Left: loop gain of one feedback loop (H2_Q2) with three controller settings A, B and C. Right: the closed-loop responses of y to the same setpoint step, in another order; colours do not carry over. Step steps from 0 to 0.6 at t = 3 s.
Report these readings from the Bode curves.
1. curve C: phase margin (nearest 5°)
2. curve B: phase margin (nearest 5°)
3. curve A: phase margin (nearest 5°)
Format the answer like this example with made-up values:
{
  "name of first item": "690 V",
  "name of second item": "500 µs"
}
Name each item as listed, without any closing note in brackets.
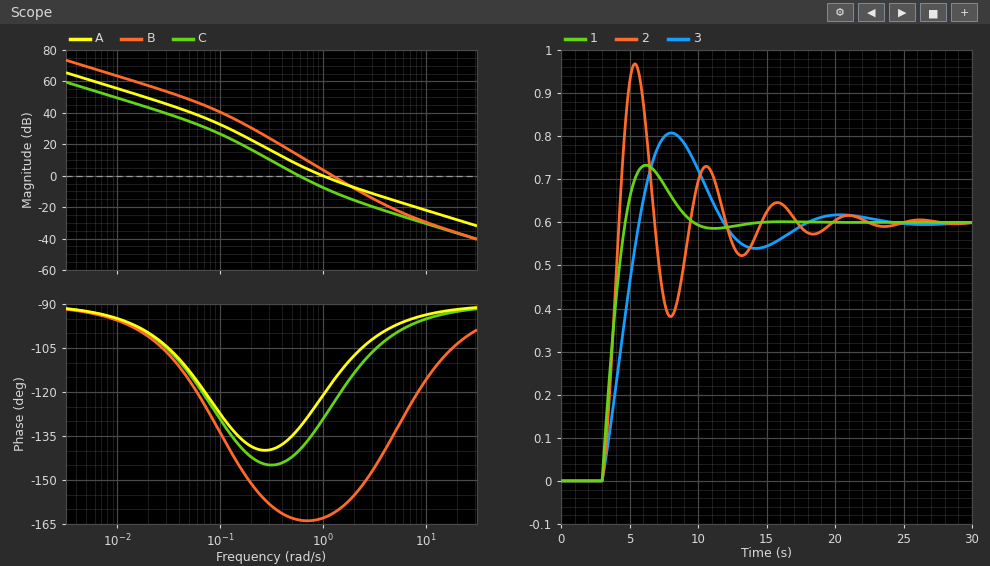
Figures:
{
  "curve C: phase margin": "40°",
  "curve B: phase margin": "20°",
  "curve A: phase margin": "60°"
}
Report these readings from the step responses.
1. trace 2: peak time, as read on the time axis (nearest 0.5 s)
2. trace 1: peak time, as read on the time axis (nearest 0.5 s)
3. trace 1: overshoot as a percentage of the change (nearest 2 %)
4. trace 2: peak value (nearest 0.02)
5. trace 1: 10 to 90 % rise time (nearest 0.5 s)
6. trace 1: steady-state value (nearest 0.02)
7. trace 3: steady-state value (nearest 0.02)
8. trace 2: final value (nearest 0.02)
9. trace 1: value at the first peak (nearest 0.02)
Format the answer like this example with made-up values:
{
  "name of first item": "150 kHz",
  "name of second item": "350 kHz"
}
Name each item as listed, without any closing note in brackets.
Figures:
{
  "trace 2: peak time, as read on the time axis": "5.5 s",
  "trace 1: peak time, as read on the time axis": "6.0 s",
  "trace 1: overshoot as a percentage of the change": "22 %",
  "trace 2: peak value": "0.96",
  "trace 1: 10 to 90 % rise time": "1.5 s",
  "trace 1: steady-state value": "0.60",
  "trace 3: steady-state value": "0.60",
  "trace 2: final value": "0.60",
  "trace 1: value at the first peak": "0.74"
}
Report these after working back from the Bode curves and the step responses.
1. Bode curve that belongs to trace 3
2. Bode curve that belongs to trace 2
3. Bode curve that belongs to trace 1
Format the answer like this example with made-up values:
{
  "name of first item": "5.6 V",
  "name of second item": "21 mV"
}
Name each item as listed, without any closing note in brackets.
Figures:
{
  "Bode curve that belongs to trace 3": "C",
  "Bode curve that belongs to trace 2": "B",
  "Bode curve that belongs to trace 1": "A"
}
